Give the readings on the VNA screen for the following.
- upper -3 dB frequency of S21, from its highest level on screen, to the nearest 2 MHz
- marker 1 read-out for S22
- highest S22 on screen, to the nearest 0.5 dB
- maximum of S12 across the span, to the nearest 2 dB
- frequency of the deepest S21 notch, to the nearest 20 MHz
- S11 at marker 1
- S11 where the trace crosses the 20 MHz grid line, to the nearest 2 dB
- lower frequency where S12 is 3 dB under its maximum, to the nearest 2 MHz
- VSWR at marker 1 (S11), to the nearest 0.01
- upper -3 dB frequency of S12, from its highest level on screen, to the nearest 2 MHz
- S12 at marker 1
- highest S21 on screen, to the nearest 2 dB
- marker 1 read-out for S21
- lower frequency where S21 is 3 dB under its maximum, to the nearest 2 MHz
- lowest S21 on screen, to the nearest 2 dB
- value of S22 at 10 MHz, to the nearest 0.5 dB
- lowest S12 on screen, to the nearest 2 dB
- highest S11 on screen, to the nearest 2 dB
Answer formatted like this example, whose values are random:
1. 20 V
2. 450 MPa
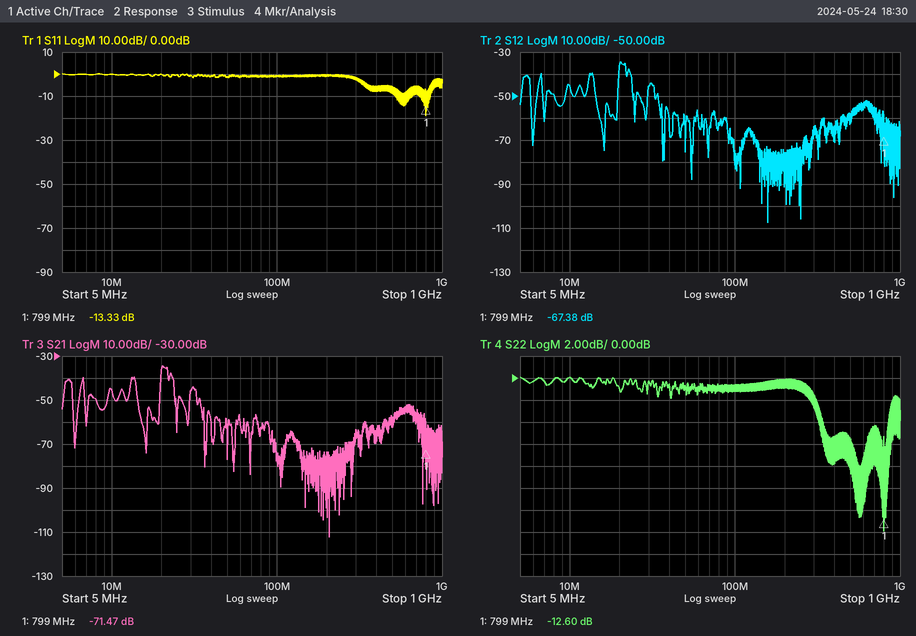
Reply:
1. 22 MHz
2. -12.60 dB
3. 0.0 dB
4. -34 dB
5. 200 MHz
6. -13.33 dB
7. 0 dB
8. 20 MHz
9. 1.55
10. 22 MHz
11. -67.38 dB
12. -34 dB
13. -71.47 dB
14. 20 MHz
15. -112 dB
16. 0.0 dB
17. -108 dB
18. 0 dB
